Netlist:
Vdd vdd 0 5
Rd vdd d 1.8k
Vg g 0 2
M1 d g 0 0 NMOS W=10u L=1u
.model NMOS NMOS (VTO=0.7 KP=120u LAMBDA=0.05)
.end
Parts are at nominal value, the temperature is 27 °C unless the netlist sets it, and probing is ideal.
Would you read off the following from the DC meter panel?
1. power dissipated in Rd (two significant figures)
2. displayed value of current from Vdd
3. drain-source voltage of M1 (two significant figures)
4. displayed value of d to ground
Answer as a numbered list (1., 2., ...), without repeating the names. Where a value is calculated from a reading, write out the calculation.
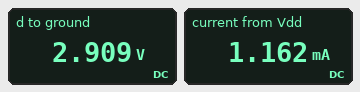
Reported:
1. (5 V - 2.909 V)^2 / 1.8 kΩ = 2.4 mW
2. 1.162 mA
3. 2.909 V = 2.9 V
4. 2.909 V
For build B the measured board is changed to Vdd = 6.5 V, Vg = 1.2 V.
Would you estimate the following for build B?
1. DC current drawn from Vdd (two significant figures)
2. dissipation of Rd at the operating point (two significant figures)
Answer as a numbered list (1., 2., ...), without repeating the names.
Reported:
1. 200 µA
2. 69 µW
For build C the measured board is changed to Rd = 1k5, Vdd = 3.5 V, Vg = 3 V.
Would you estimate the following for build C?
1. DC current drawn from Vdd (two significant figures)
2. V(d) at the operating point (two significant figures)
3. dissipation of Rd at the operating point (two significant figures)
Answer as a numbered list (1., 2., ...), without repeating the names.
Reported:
1. 1.8 mA
2. 760 mV
3. 5.0 mW
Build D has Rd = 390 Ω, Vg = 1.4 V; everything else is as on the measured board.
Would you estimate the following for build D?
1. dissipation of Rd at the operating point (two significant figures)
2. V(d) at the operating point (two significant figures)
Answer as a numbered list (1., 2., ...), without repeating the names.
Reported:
1. 52 µW
2. 4.9 V
